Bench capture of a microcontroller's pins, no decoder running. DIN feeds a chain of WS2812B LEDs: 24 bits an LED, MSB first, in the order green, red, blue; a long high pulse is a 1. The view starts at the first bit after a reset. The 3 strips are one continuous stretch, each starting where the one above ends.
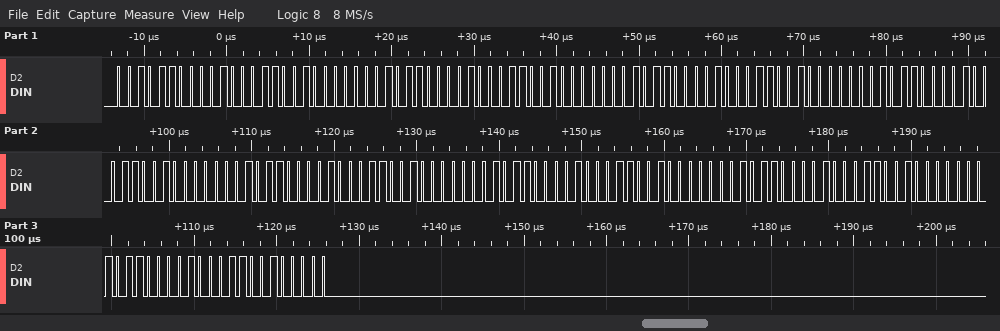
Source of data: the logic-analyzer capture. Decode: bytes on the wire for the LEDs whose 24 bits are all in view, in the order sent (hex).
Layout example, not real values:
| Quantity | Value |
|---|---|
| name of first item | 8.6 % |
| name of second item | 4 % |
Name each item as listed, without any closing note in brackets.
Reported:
| Quantity | Value |
|---|---|
| bytes on the wire for the LEDs whose 24 bits are all in view, in the order sent | 2C 23 20 2C 23 20 2C 23 20 2C 23 20 2C 23 20 2C 23 20 2C 23 20 2C 23 20 |
